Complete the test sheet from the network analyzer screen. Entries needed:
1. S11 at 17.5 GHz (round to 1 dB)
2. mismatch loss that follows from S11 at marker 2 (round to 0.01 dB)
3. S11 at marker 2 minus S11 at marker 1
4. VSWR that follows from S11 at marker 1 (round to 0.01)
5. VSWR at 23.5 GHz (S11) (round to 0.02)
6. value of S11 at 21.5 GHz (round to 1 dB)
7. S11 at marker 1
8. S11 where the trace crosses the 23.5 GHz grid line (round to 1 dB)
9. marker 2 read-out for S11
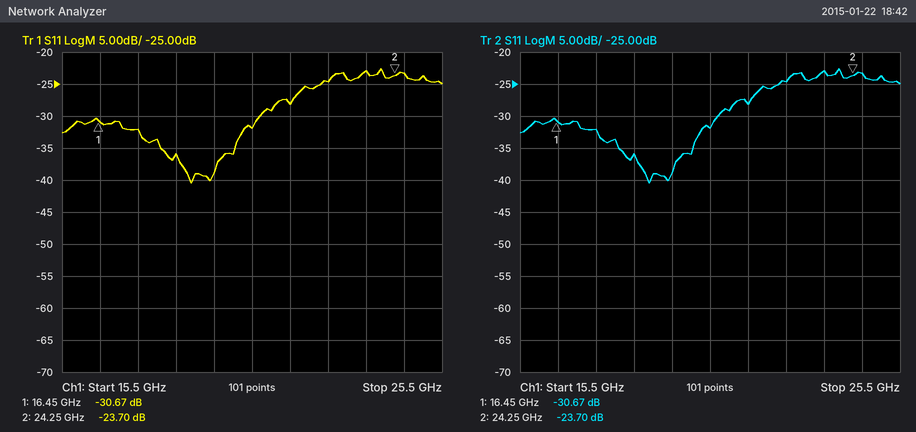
-32 dB
0.02 dB
6.97 dB
1.06
1.16
-28 dB
-30.67 dB
-23 dB
-23.70 dB
